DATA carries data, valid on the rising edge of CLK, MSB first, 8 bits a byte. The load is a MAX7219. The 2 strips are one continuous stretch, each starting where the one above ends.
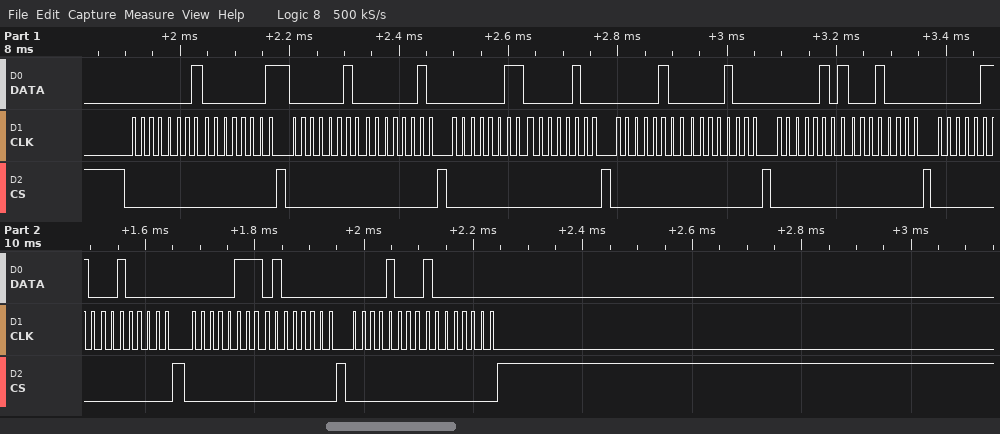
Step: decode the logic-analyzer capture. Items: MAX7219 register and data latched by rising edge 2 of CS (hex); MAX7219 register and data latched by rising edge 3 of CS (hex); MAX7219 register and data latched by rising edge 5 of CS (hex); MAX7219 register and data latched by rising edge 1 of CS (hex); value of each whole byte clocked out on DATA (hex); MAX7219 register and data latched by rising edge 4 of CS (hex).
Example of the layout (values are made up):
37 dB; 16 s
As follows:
register 0x2, data 0x02; register 0x3, data 0x04; register 0x5, data 0x10; register 0x1, data 0x01; 0x01 0x01 0x02 0x02 0x03 0x04 0x04 0x08 0x05 0x10 0x06 0x20 0x07 0x40 0x08 0x80; register 0x4, data 0x08
